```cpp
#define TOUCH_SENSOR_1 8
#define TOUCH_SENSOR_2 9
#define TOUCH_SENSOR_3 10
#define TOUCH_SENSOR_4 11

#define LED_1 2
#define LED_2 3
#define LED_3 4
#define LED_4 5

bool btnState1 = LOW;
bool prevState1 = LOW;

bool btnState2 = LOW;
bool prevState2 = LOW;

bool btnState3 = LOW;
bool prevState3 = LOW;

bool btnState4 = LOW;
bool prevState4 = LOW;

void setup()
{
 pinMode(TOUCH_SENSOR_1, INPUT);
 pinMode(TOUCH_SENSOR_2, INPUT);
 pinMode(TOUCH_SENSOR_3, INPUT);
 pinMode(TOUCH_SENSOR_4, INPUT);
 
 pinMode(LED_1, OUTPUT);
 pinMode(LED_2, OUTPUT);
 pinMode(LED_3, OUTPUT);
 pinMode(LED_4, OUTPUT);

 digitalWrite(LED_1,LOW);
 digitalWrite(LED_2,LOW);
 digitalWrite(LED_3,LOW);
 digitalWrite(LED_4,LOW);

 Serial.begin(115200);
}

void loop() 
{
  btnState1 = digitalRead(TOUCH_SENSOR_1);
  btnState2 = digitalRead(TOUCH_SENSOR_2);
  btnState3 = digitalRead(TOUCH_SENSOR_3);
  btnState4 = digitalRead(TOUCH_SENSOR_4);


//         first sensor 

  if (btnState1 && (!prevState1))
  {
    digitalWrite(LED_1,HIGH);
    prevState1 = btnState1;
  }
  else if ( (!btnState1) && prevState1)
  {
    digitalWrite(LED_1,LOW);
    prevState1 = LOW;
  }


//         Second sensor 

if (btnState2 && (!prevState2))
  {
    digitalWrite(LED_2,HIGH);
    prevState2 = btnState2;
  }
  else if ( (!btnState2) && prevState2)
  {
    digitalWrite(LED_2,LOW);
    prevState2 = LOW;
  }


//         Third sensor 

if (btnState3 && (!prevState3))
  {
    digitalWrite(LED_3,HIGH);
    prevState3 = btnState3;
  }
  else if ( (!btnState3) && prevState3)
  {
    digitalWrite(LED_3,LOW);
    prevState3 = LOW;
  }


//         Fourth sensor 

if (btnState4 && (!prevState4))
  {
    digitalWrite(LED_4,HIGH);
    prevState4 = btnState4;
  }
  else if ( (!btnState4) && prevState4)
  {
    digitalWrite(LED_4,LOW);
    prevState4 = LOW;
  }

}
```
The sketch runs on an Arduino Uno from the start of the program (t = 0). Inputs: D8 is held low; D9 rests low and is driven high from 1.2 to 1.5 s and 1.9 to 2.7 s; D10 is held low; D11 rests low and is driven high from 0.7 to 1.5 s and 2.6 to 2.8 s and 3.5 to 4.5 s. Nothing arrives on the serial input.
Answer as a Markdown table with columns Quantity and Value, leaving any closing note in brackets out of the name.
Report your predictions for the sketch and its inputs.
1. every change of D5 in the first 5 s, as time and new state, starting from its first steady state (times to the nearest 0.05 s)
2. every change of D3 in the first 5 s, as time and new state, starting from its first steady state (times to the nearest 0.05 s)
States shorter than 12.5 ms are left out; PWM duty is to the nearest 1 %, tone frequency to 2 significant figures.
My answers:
| Quantity | Value |
|---|---|
| every change of D5 in the first 5 s, as time and new state, starting from its first steady state | 0 s low; 0.7 s high; 1.5 s low; 2.6 s high; 2.8 s low; 3.5 s high; 4.5 s low |
| every change of D3 in the first 5 s, as time and new state, starting from its first steady state | 0 s low; 1.2 s high; 1.5 s low; 1.9 s high; 2.7 s low |
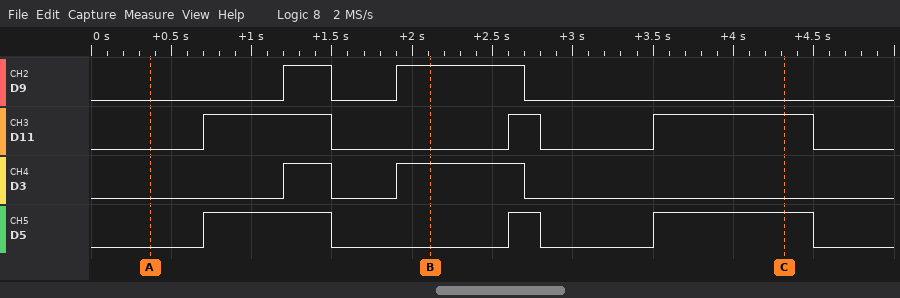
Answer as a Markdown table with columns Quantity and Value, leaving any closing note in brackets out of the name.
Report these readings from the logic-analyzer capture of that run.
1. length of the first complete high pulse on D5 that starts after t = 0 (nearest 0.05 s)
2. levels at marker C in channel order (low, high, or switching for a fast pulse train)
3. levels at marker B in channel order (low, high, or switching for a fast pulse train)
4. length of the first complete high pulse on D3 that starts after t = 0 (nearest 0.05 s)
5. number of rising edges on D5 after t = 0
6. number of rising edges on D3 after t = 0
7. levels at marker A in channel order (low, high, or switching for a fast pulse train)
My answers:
| Quantity | Value |
|---|---|
| length of the first complete high pulse on D5 that starts after t = 0 | 0.80 s |
| levels at marker C in channel order | D9 low, D11 high, D3 low, D5 high |
| levels at marker B in channel order | D9 high, D11 low, D3 high, D5 low |
| length of the first complete high pulse on D3 that starts after t = 0 | 0.30 s |
| number of rising edges on D5 after t = 0 | 3 |
| number of rising edges on D3 after t = 0 | 2 |
| levels at marker A in channel order | D9 low, D11 low, D3 low, D5 low |
